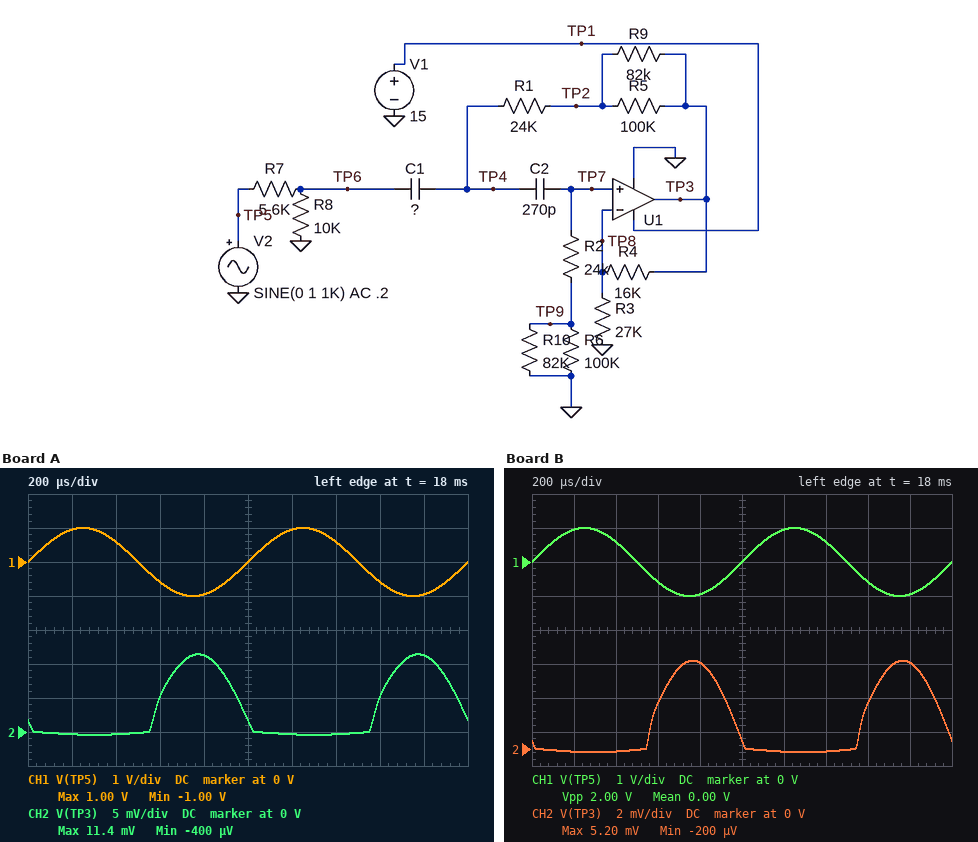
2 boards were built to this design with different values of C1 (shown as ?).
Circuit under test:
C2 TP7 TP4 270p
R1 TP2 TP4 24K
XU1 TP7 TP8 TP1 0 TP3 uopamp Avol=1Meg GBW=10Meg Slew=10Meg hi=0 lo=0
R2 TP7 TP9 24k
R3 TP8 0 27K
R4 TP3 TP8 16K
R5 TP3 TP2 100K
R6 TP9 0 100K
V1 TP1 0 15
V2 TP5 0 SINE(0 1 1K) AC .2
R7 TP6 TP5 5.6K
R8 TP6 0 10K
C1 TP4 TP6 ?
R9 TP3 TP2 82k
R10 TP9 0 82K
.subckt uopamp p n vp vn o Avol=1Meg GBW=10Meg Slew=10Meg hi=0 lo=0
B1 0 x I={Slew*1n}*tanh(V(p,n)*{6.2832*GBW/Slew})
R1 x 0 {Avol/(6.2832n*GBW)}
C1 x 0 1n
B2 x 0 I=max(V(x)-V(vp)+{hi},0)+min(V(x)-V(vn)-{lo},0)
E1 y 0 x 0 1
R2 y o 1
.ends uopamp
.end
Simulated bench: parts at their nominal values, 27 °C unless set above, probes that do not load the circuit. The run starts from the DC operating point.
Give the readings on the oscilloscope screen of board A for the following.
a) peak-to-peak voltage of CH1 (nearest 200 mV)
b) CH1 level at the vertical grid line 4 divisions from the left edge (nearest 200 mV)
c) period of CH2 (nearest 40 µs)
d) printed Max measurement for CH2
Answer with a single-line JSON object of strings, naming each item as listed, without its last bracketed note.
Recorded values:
{"peak-to-peak voltage of CH1": "2.0 V", "CH1 level at the vertical grid line 4 divisions from the left edge": "-1.0 V", "period of CH2": "1.00 ms", "printed Max measurement for CH2": "11.4 mV"}
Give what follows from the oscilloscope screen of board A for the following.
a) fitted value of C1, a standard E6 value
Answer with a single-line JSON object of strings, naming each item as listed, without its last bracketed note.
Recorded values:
{"fitted value of C1, a standard E6 value": "220 pF"}
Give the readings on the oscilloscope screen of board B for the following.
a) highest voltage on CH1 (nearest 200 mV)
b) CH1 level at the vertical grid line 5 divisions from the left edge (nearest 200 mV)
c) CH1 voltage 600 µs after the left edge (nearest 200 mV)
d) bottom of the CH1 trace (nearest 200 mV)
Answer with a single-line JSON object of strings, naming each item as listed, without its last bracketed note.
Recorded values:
{"highest voltage on CH1": "1.0 V", "CH1 level at the vertical grid line 5 divisions from the left edge": "0 V", "CH1 voltage 600 µs after the left edge": "-600 mV", "bottom of the CH1 trace": "-1.0 V"}
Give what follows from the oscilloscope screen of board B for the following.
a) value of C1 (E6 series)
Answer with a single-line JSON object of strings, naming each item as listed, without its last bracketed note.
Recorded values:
{"value of C1": "100 pF"}
